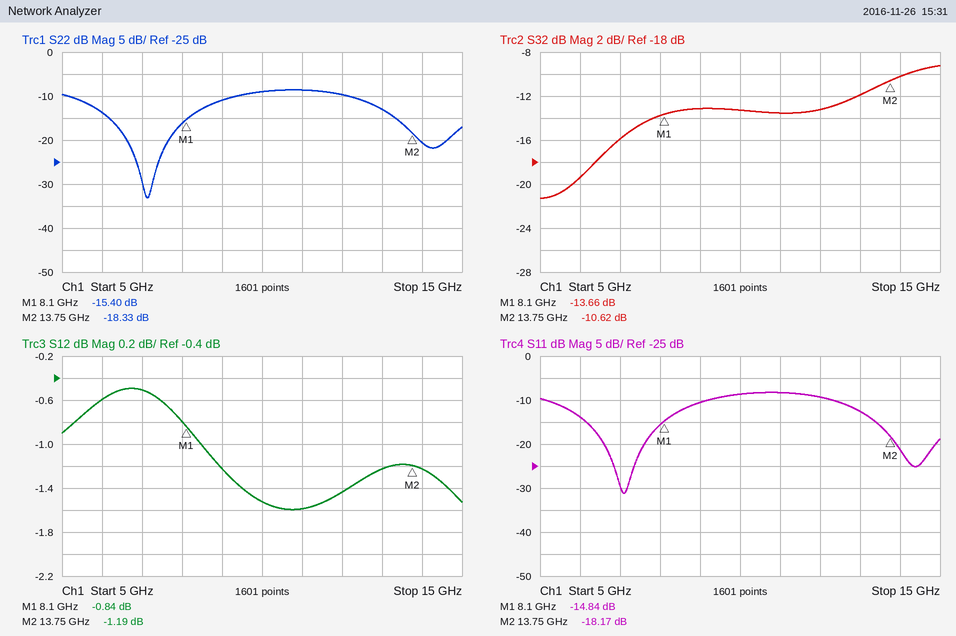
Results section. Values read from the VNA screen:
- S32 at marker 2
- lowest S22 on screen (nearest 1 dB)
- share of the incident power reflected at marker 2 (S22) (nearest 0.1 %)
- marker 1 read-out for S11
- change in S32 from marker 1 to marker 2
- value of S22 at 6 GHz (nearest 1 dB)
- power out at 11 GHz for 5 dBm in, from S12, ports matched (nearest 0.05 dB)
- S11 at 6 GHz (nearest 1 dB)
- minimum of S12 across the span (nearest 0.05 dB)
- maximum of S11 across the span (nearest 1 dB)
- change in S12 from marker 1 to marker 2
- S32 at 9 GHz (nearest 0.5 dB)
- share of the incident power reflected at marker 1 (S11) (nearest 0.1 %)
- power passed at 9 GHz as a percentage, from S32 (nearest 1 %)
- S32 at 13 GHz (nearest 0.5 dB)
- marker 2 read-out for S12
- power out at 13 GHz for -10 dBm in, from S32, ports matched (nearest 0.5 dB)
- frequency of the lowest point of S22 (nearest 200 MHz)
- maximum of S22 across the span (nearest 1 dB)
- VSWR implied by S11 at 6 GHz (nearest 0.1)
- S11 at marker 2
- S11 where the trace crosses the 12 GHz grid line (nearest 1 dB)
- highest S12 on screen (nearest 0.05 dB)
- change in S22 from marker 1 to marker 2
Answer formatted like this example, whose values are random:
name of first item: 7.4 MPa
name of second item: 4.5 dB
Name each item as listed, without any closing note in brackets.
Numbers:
S32 at marker 2: -10.62 dB
lowest S22 on screen: -33 dB
share of the incident power reflected at marker 2 (S22): 1.5 %
marker 1 read-out for S11: -14.84 dB
change in S32 from marker 1 to marker 2: 3.04 dB
value of S22 at 6 GHz: -14 dB
power out at 11 GHz for 5 dBm in, from S12, ports matched: 3.40 dBm
S11 at 6 GHz: -14 dB
minimum of S12 across the span: -1.60 dB
maximum of S11 across the span: -8 dB
change in S12 from marker 1 to marker 2: -0.35 dB
S32 at 9 GHz: -13.0 dB
share of the incident power reflected at marker 1 (S11): 3.3 %
power passed at 9 GHz as a percentage, from S32: 5 %
S32 at 13 GHz: -12.0 dB
marker 2 read-out for S12: -1.19 dB
power out at 13 GHz for -10 dBm in, from S32, ports matched: -22.0 dBm
frequency of the lowest point of S22: 7.2 GHz
maximum of S22 across the span: -9 dB
VSWR implied by S11 at 6 GHz: 1.5
S11 at marker 2: -18.17 dB
S11 where the trace crosses the 12 GHz grid line: -9 dB
highest S12 on screen: -0.50 dB
change in S22 from marker 1 to marker 2: -2.93 dB
